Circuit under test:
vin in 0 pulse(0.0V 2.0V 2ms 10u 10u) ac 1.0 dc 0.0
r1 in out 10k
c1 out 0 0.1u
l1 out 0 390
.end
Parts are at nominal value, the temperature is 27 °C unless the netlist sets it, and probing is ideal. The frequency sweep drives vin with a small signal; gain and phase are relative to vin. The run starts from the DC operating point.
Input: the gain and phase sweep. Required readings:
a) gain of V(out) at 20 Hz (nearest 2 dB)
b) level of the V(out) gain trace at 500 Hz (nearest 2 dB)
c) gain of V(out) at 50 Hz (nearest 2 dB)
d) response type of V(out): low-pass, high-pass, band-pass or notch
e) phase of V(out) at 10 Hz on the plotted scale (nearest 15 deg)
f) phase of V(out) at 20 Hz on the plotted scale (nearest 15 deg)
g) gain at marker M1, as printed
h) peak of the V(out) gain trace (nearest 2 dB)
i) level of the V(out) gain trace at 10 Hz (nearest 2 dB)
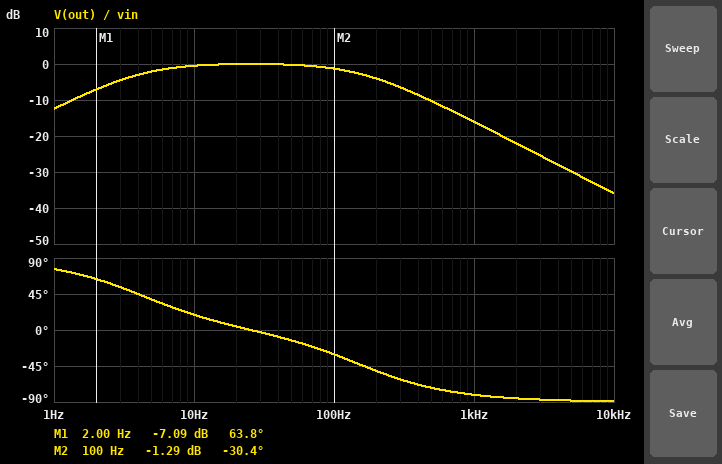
0 dB
-10 dB
0 dB
band-pass
15 deg
0 deg
-7.09 dB
0 dB
0 dB
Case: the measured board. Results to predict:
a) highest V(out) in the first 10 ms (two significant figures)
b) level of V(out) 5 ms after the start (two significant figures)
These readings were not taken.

1.9 V
1.8 V
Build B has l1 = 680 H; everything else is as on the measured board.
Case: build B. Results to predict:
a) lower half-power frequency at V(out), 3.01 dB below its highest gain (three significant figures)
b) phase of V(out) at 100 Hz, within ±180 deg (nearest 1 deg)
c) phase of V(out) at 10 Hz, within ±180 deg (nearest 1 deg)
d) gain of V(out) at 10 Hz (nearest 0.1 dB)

2.31 Hz
-31 deg
10 deg
-0.1 dB
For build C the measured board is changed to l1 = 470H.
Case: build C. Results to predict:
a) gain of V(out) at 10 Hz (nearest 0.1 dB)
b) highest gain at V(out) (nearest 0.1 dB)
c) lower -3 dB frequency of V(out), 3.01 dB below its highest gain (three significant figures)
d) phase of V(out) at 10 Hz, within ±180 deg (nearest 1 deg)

-0.3 dB
0 dB
3.32 Hz
15 deg
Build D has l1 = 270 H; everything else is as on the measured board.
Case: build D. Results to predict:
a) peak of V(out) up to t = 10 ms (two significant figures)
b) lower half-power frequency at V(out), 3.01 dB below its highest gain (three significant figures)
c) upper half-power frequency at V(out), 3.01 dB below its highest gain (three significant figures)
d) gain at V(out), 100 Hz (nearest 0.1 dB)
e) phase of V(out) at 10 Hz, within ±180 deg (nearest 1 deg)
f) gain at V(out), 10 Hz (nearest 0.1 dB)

1.8 V
5.69 Hz
165 Hz
-1.2 dB
28 deg
-1.1 dB
